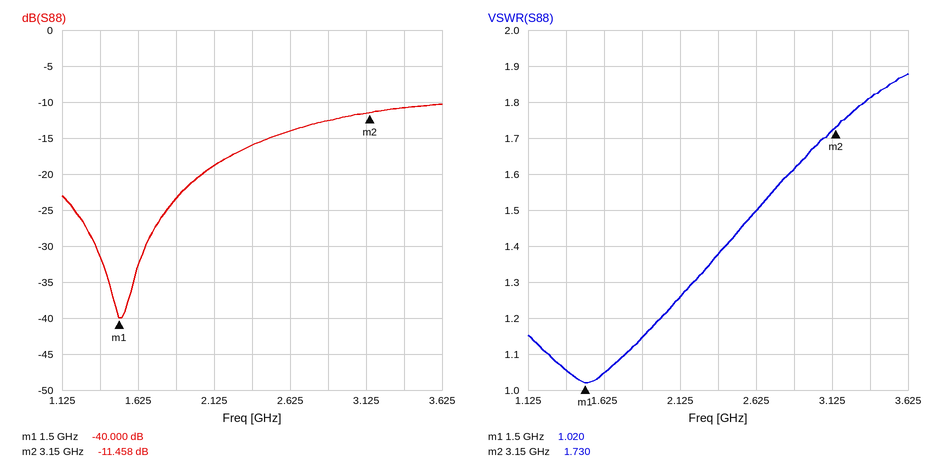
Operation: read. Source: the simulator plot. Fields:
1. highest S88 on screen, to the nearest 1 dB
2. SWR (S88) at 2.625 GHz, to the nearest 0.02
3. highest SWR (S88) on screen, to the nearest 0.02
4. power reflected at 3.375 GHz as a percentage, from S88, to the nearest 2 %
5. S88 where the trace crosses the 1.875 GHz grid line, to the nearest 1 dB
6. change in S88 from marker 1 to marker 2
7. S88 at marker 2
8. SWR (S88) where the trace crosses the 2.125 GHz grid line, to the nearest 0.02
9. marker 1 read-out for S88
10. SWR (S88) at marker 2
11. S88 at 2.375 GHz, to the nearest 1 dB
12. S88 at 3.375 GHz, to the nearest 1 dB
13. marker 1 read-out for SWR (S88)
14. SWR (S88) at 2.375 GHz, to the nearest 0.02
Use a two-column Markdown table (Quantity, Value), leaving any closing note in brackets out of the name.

| Quantity | Value |
|---|---|
| highest S88 on screen, to the nearest 1 dB | -10 dB |
| SWR (S88) at 2.625 GHz, to the nearest 0.02 | 1.50 |
| highest SWR (S88) on screen, to the nearest 0.02 | 1.88 |
| power reflected at 3.375 GHz as a percentage, from S88, to the nearest 2 % | 8 % |
| S88 where the trace crosses the 1.875 GHz grid line, to the nearest 1 dB | -23 dB |
| change in S88 from marker 1 to marker 2 | 28.542 dB |
| S88 at marker 2 | -11.458 dB |
| SWR (S88) where the trace crosses the 2.125 GHz grid line, to the nearest 0.02 | 1.26 |
| marker 1 read-out for S88 | -40.000 dB |
| SWR (S88) at marker 2 | 1.730 |
| S88 at 2.375 GHz, to the nearest 1 dB | -16 dB |
| S88 at 3.375 GHz, to the nearest 1 dB | -11 dB |
| marker 1 read-out for SWR | 1.020 |
| SWR (S88) at 2.375 GHz, to the nearest 0.02 | 1.38 |
